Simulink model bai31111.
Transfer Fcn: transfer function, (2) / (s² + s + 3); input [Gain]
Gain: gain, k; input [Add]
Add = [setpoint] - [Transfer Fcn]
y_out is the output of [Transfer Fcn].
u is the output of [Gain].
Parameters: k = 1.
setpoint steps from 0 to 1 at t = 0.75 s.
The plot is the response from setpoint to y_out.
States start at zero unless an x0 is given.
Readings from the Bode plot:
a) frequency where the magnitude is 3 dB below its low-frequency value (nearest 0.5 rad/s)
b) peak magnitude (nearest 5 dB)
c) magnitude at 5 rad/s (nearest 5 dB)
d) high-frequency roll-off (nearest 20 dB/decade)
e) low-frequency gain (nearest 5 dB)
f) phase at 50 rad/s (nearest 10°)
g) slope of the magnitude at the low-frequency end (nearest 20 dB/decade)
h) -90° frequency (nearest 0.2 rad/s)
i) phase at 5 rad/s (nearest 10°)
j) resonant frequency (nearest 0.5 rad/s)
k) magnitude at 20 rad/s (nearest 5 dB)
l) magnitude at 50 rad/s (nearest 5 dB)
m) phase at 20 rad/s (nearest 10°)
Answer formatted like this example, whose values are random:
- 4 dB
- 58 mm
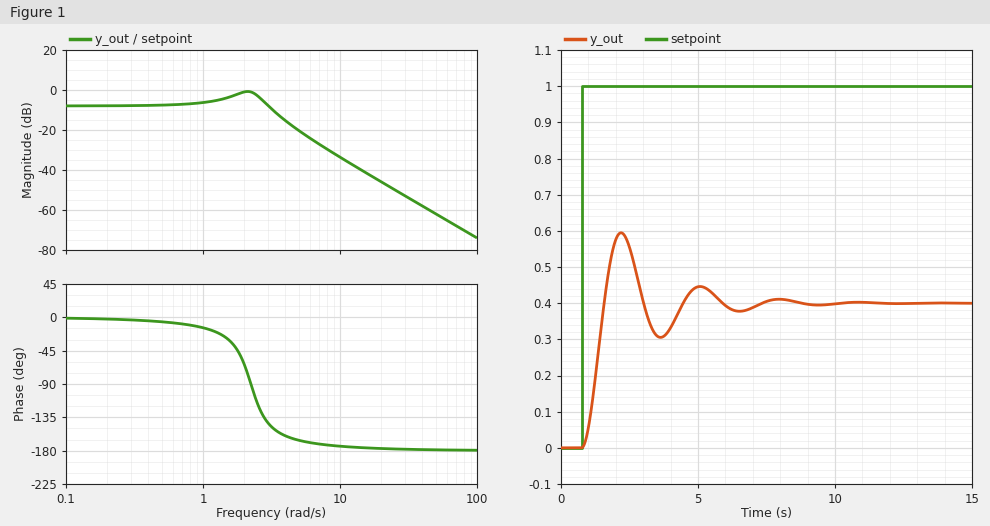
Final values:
- 3.5 rad/s
- 0 dB
- -20 dB
- -40 dB/decade
- -10 dB
- -180°
- 0 dB/decade
- 2.2 rad/s
- -170°
- 2.0 rad/s
- -45 dB
- -60 dB
- -180°
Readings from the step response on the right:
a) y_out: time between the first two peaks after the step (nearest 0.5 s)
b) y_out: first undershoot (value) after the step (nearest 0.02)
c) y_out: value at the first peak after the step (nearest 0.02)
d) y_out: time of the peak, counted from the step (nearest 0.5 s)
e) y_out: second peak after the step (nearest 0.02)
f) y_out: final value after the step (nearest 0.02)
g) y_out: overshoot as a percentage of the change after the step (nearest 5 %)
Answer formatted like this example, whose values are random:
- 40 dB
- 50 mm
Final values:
- 3.0 s
- 0.30
- 0.60
- 1.5 s
- 0.44
- 0.40
- 50 %
